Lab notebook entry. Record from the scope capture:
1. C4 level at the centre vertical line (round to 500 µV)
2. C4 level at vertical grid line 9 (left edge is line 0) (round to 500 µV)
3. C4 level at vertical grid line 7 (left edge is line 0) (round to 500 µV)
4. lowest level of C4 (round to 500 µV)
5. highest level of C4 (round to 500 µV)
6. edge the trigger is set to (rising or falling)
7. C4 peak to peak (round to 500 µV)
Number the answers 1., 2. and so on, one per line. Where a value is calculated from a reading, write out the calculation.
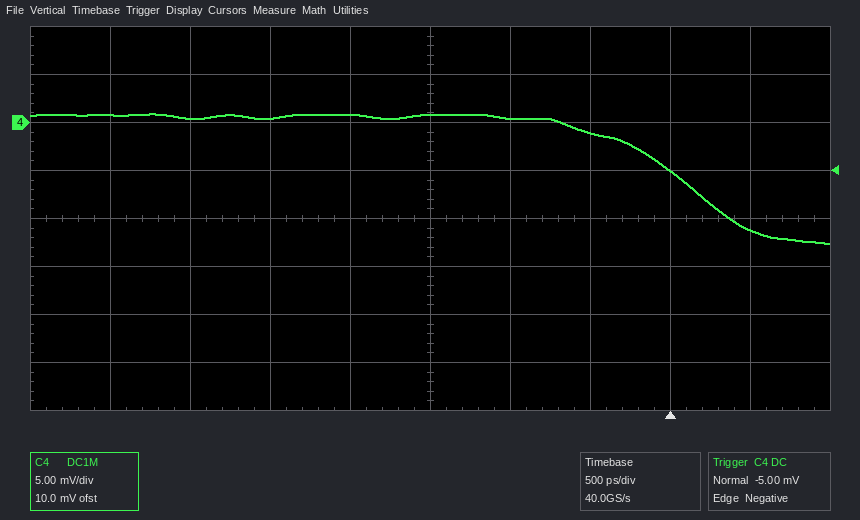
1. 1.0 mV
2. -11.0 mV
3. -1.0 mV
4. -12.5 mV
5. 1.0 mV
6. falling
7. 1.0 mV − (-12.5 mV) = 13.5 mV
